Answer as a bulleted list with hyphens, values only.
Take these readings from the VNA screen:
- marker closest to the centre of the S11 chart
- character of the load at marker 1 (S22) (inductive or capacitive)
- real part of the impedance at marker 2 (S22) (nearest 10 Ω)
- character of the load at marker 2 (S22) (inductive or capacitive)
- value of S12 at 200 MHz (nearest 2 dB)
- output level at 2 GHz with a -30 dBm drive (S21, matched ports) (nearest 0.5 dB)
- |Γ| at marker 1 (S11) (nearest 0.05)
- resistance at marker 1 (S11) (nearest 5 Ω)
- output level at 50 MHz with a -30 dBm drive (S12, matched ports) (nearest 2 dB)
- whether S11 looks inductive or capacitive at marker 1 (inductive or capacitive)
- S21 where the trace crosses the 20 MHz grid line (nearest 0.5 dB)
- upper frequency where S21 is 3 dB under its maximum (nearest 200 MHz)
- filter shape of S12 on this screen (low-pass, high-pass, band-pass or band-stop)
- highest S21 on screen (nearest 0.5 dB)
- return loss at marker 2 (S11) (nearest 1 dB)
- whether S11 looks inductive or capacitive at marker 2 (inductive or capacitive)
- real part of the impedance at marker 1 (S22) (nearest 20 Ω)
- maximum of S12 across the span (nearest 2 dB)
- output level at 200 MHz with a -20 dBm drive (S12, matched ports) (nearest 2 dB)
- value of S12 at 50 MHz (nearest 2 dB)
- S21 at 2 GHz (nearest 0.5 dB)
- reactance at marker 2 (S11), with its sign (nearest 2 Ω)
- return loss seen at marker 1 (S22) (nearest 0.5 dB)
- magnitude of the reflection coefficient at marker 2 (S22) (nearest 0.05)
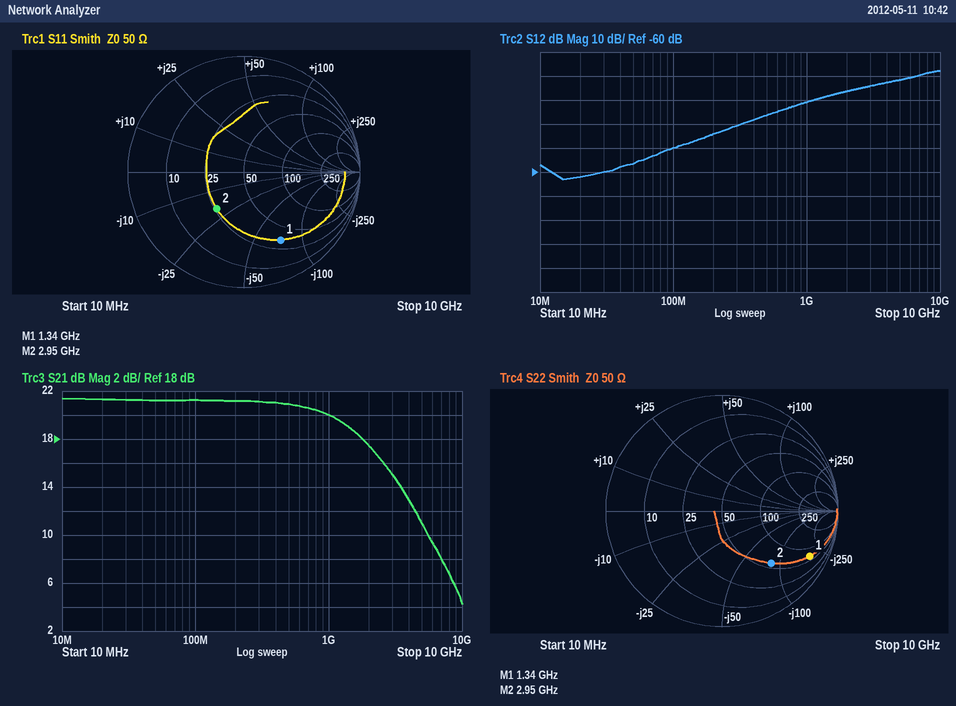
- marker 2
- capacitive
- 60 Ω
- capacitive
- -44 dB
- -12.5 dBm
- 0.65
- 35 Ω
- -86 dBm
- capacitive
- 21.5 dB
- 1.6 GHz
- high-pass
- 21.5 dB
- 8 dB
- capacitive
- 60 Ω
- -18 dB
- -64 dBm
- -56 dB
- 17.5 dB
- -20 Ω
- 1.5 dB
- 0.60
